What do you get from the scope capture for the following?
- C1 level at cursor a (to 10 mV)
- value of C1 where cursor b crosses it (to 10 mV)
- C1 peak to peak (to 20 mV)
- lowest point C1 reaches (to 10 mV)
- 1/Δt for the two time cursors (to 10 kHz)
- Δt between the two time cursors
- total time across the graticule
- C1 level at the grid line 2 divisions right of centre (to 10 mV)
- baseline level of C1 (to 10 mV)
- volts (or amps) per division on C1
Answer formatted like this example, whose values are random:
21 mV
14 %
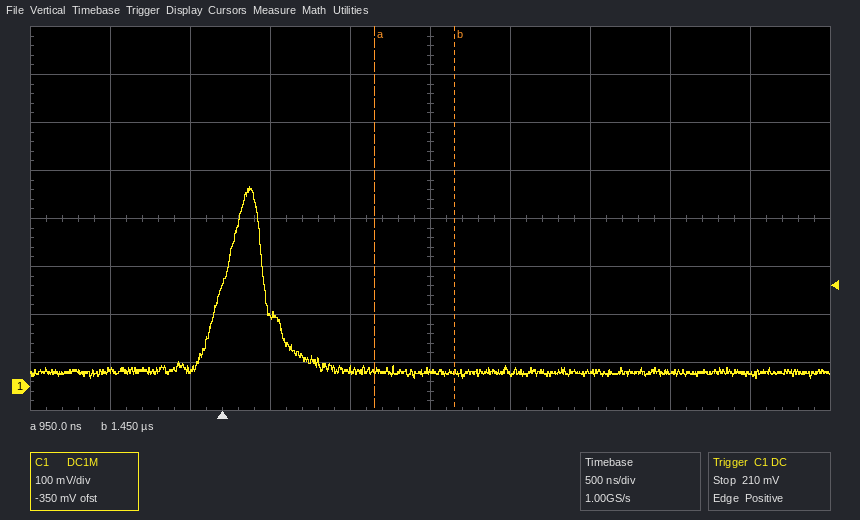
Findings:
30 mV
30 mV
400 mV
20 mV
2.00 MHz
500 ns
5 µs
30 mV
30 mV
100 mV
